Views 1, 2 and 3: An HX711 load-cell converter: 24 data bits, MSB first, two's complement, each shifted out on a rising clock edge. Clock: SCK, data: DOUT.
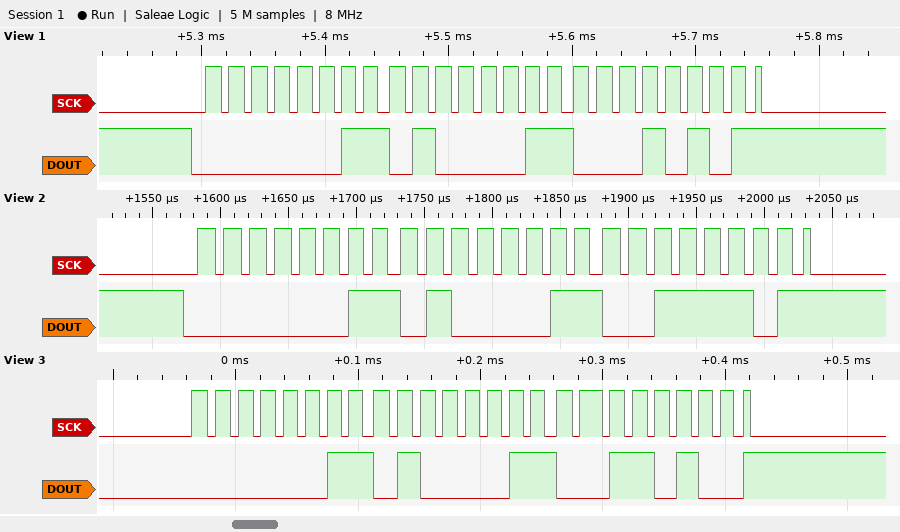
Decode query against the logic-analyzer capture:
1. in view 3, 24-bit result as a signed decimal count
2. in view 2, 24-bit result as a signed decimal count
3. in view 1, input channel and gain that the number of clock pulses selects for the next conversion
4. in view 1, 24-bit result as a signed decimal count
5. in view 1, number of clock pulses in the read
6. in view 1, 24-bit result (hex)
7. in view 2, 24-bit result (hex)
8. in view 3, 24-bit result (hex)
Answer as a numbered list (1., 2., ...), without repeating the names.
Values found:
1. 213812
2. 213821
3. channel A, gain 128
4. 213781
5. 25
6. 0x034315
7. 0x03433D
8. 0x034334
